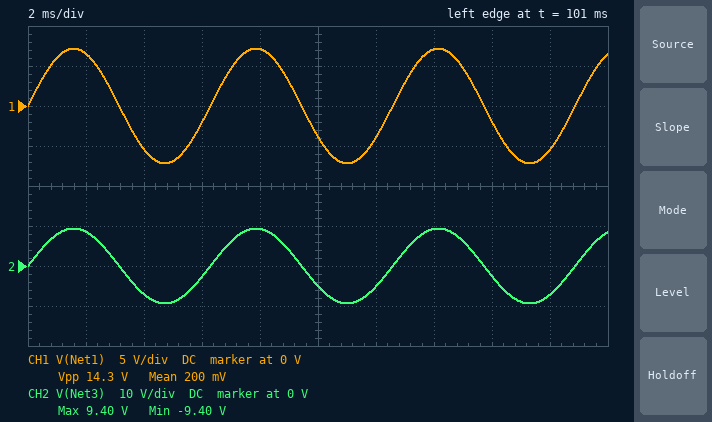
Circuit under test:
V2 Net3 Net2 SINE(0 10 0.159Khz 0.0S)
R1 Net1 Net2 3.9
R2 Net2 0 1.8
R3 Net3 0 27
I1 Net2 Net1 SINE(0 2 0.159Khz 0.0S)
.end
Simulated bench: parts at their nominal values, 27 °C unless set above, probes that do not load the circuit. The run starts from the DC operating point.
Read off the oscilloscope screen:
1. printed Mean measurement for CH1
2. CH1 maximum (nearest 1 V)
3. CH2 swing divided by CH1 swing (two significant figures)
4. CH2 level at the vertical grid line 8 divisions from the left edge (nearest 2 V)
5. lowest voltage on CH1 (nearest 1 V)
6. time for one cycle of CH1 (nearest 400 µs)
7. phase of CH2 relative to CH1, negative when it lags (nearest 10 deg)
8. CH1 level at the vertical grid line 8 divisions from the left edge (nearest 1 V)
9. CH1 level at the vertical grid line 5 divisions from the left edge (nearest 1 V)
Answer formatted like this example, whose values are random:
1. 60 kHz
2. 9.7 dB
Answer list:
1. 200 mV
2. 7 V
3. 1.3
4. -2 V
5. -7 V
6. 6.4 ms
7. 0 deg
8. -2 V
9. -4 V
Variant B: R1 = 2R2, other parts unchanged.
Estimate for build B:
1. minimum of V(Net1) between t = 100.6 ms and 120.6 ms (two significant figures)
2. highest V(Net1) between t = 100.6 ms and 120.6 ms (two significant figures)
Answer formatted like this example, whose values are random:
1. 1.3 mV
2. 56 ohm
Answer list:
1. -3.8 V
2. 3.8 V
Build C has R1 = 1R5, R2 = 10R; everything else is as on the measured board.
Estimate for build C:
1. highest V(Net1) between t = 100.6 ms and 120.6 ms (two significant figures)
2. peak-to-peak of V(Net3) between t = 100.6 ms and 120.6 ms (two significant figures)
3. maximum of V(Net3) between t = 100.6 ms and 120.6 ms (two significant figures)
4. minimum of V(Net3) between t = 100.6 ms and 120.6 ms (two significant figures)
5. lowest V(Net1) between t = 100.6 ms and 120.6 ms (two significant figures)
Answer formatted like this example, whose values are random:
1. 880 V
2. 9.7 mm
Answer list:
1. 300 mV
2. 15 V
3. 7.3 V
4. -7.3 V
5. -300 mV
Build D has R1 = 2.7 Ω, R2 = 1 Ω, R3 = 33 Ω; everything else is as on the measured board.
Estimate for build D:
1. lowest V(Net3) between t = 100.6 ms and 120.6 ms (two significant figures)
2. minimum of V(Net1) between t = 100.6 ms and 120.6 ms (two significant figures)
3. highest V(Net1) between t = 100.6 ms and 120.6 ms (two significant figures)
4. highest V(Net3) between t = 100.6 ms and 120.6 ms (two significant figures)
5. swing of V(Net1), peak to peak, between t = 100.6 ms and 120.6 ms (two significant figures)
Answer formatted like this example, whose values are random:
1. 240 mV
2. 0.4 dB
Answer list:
1. -9.7 V
2. -5.1 V
3. 5.1 V
4. 9.7 V
5. 10 V
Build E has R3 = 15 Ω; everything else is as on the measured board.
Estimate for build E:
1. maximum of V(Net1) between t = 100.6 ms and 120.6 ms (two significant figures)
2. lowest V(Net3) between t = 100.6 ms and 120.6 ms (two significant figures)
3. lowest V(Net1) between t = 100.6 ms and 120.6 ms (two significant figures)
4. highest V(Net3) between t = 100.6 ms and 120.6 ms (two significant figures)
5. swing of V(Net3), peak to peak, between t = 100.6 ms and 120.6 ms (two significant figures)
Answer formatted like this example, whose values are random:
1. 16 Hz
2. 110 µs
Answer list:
1. 6.7 V
2. -8.9 V
3. -6.7 V
4. 8.9 V
5. 18 V
